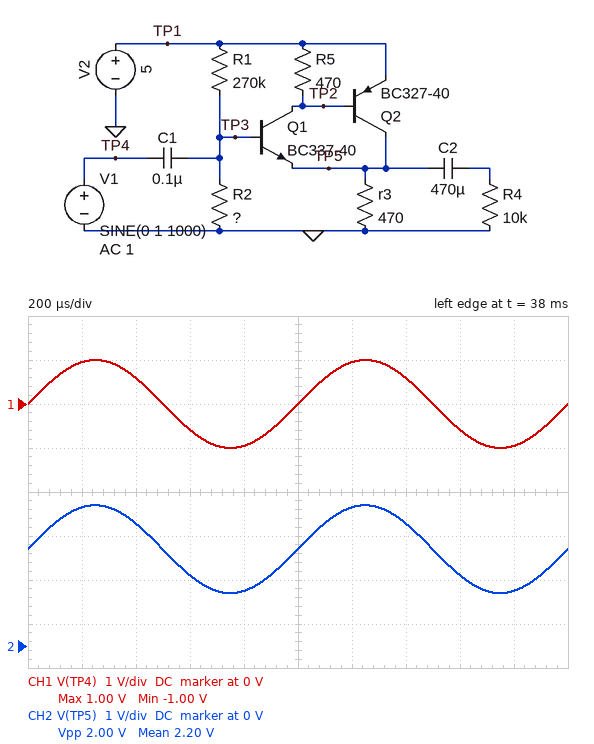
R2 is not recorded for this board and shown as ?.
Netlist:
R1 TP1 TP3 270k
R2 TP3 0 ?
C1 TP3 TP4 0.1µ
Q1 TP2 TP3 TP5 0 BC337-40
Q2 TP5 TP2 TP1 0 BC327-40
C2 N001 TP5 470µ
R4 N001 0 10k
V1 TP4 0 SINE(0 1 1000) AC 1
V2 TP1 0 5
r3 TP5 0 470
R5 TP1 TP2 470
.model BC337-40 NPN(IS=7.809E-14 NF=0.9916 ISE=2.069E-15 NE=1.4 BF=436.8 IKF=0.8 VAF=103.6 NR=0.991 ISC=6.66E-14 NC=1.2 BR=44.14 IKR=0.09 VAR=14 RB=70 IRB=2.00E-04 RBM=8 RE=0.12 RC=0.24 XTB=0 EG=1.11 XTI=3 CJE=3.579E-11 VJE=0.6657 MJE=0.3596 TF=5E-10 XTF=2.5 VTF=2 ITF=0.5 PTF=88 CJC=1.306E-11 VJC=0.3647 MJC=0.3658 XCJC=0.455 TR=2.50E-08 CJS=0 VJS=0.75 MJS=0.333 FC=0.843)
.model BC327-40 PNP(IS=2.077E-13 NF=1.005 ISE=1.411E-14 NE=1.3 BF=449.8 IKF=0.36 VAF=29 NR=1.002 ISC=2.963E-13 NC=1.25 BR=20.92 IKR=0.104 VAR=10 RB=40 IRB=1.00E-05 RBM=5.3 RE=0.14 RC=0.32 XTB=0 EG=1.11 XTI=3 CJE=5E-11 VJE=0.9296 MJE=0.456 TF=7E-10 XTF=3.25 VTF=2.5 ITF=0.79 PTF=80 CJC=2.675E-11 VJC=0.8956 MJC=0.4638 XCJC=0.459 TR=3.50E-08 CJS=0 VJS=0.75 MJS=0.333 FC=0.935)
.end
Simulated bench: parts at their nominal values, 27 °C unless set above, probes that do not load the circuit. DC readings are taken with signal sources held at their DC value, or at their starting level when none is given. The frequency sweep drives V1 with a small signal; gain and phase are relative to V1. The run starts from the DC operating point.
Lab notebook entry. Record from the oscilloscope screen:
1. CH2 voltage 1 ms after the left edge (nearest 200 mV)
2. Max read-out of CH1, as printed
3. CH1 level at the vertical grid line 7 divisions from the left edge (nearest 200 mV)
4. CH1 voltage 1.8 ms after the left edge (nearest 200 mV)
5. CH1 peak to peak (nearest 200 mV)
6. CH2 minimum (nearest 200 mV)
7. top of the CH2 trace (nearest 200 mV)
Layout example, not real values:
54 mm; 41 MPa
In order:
2.2 V; 1.00 V; 600 mV; -1.0 V; 2.0 V; 1.2 V; 3.2 V
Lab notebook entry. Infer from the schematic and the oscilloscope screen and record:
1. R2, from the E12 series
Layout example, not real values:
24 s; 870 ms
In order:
560 kΩ
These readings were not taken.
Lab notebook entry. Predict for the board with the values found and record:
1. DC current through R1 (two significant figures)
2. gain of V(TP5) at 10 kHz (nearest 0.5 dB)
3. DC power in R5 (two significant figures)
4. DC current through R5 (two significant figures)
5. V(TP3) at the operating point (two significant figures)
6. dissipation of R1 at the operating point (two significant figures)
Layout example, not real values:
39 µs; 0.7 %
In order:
8.1 µA; 0 dB; 800 µW; 1.3 mA; 2.8 V; 18 µW
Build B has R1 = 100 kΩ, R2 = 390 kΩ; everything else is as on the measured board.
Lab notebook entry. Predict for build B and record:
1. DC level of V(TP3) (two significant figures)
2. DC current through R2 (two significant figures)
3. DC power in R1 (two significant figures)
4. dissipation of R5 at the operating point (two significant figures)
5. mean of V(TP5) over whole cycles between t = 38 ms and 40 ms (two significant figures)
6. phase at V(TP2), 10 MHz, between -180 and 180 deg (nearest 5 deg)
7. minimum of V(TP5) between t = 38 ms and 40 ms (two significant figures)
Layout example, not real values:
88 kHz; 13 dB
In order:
3.7 V; 9.5 µA; 16 µW; 830 µW; 3.1 V; -145 deg; 2.1 V
